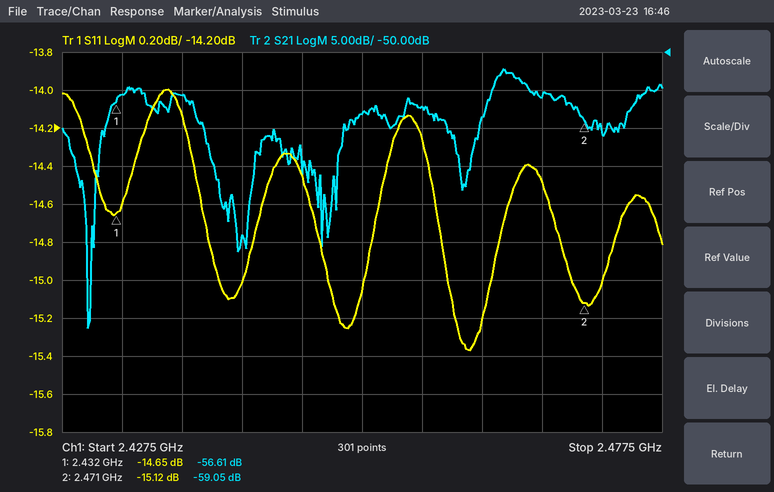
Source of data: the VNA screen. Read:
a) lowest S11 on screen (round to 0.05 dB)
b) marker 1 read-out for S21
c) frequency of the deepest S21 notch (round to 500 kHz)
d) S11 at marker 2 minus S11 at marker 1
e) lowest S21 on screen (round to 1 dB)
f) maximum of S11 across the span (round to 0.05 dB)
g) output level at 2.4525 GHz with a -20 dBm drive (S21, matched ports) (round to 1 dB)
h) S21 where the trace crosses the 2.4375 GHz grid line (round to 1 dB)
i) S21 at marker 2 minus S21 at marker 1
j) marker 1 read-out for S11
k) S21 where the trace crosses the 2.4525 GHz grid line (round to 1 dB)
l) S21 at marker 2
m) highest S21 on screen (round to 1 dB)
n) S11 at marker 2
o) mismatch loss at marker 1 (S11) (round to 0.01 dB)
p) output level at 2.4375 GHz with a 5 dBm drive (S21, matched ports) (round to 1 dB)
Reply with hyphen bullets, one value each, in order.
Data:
- -15.35 dB
- -56.61 dB
- 2.4295 GHz
- -0.47 dB
- -86 dB
- -14.00 dB
- -78 dBm
- -56 dB
- -2.44 dB
- -14.65 dB
- -58 dB
- -59.05 dB
- -52 dB
- -15.12 dB
- 0.15 dB
- -51 dBm
